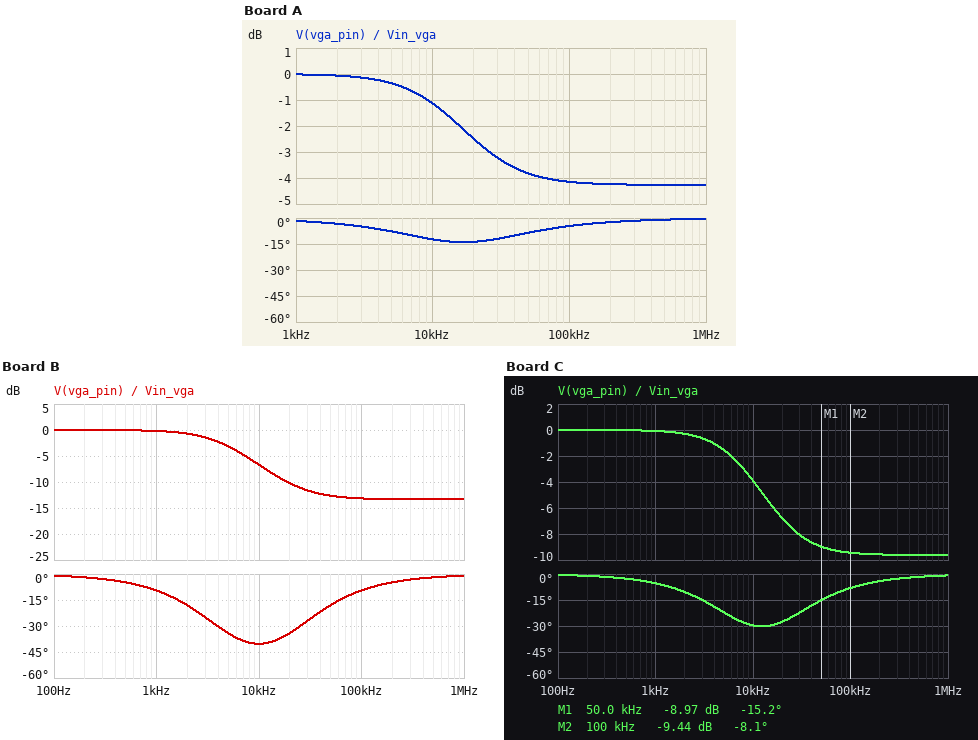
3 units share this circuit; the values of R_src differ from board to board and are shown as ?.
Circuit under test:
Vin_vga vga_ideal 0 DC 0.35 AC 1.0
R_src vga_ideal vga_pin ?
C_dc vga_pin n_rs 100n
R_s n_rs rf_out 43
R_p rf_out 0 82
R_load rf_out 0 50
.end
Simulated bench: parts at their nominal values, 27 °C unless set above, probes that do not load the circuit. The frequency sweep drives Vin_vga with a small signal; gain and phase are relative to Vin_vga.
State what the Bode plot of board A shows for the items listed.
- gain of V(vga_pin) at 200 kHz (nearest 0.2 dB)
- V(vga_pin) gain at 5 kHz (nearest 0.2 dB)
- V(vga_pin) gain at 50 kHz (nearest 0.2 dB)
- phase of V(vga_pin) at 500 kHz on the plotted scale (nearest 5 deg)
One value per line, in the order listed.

-4.2 dB
-0.4 dB
-3.8 dB
0 deg
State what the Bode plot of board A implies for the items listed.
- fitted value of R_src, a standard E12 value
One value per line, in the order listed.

47 Ω
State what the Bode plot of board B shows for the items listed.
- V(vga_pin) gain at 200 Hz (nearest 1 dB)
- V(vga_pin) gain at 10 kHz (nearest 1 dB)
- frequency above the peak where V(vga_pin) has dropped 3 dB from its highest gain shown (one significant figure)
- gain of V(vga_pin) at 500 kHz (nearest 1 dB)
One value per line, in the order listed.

0 dB
-7 dB
5 kHz
-13 dB
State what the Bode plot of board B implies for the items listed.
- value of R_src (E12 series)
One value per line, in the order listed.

270 Ω
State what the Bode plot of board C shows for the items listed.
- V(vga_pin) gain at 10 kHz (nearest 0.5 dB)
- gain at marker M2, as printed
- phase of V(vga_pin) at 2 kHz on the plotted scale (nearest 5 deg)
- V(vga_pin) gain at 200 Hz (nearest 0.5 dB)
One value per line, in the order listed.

-4.0 dB
-9.44 dB
-10 deg
0 dB
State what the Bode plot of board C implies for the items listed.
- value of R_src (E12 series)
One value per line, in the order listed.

150 Ω
